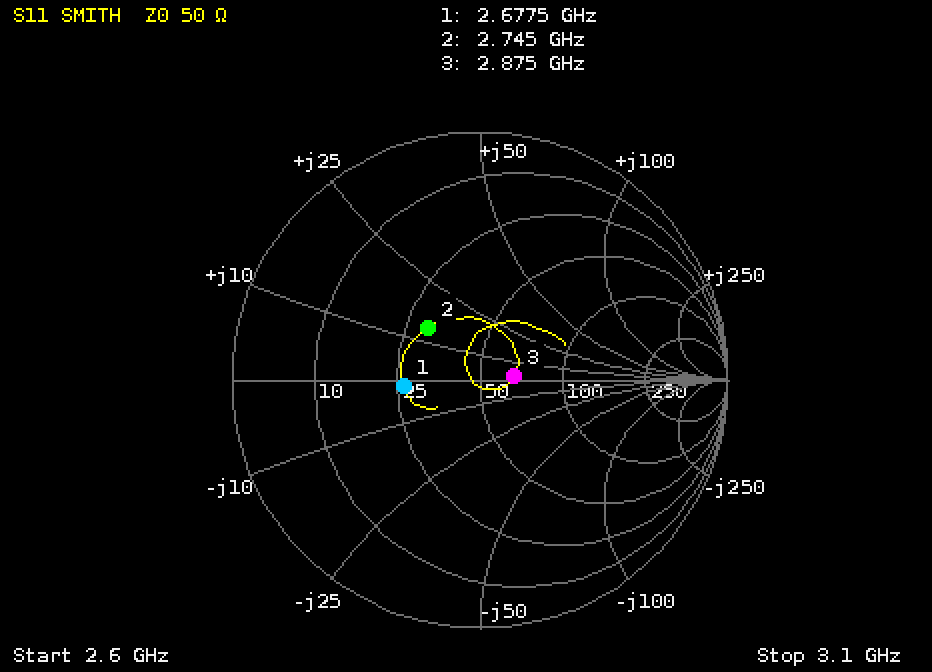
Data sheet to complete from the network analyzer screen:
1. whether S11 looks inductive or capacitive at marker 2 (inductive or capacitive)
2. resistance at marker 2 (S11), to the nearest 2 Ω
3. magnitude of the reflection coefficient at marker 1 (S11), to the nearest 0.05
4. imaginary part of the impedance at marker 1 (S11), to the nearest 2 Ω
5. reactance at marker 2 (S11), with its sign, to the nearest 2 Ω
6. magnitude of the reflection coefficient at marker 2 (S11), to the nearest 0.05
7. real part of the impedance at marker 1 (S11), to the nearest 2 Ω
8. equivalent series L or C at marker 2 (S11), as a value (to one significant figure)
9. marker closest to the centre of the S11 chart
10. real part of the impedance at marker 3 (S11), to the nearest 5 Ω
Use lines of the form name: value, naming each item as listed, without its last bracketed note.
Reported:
whether S11 looks inductive or capacitive at marker 2: inductive
resistance at marker 2 (S11), to the nearest 2 Ω: 30 Ω
magnitude of the reflection coefficient at marker 1 (S11), to the nearest 0.05: 0.30
imaginary part of the impedance at marker 1 (S11), to the nearest 2 Ω: -2 Ω
reactance at marker 2 (S11), with its sign, to the nearest 2 Ω: +14 Ω
magnitude of the reflection coefficient at marker 2 (S11), to the nearest 0.05: 0.30
real part of the impedance at marker 1 (S11), to the nearest 2 Ω: 26 Ω
equivalent series L or C at marker 2 (S11), as a value: 800 pH
marker closest to the centre of the S11 chart: marker 3
real part of the impedance at marker 3 (S11), to the nearest 5 Ω: 65 Ω
